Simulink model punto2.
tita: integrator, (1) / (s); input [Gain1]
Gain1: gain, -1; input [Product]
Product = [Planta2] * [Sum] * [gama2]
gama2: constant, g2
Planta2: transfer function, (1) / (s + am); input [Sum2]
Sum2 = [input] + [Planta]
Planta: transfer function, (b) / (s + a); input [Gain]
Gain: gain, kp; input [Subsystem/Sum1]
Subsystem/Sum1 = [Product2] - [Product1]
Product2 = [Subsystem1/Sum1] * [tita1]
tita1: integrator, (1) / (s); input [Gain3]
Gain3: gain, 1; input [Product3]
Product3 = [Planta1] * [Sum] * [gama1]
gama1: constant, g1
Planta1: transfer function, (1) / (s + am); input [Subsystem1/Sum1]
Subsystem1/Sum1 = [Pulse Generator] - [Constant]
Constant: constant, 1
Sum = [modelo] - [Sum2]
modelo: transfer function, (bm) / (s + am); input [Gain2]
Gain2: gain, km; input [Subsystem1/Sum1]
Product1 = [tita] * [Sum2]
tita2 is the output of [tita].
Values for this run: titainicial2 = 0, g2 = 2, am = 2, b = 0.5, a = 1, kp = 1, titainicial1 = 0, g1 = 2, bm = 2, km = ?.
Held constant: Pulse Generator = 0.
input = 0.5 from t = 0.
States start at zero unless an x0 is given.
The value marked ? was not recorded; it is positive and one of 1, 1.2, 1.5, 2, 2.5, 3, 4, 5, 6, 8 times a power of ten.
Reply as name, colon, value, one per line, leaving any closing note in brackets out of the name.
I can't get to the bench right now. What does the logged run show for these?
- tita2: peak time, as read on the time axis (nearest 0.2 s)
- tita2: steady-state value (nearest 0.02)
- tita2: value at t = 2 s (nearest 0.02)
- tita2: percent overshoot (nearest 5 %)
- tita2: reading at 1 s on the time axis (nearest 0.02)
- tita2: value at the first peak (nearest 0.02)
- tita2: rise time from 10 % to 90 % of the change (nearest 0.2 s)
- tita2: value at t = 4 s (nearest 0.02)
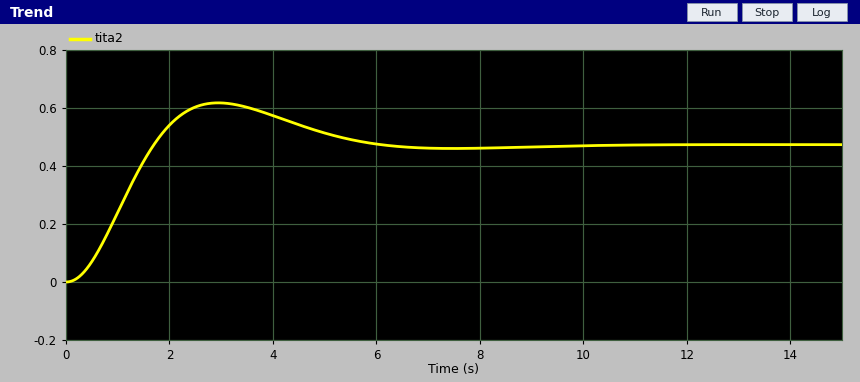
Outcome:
tita2: peak time, as read on the time axis: 3.0 s
tita2: steady-state value: 0.48
tita2: value at t = 2 s: 0.54
tita2: percent overshoot: 30 %
tita2: reading at 1 s on the time axis: 0.24
tita2: value at the first peak: 0.62
tita2: rise time from 10 % to 90 % of the change: 1.2 s
tita2: value at t = 4 s: 0.58
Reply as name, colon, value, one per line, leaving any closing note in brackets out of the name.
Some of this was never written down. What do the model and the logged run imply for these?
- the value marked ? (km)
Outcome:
the value marked ?: 0.6
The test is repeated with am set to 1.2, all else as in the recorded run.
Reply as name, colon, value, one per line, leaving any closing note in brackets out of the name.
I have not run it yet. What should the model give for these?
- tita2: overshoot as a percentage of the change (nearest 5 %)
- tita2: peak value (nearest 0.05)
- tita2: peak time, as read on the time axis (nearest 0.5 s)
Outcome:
tita2: overshoot as a percentage of the change: 25 %
tita2: peak value: 0.90
tita2: peak time, as read on the time axis: 2.5 s
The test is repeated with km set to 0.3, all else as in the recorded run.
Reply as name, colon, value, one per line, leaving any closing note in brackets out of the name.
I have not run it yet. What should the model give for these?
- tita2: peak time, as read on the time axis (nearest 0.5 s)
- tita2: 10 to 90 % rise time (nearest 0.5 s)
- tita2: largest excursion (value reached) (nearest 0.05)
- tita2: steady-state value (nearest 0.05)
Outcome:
tita2: peak time, as read on the time axis: 3.5 s
tita2: 10 to 90 % rise time: 1.5 s
tita2: largest excursion (value reached): 0.50
tita2: steady-state value: 0.50
